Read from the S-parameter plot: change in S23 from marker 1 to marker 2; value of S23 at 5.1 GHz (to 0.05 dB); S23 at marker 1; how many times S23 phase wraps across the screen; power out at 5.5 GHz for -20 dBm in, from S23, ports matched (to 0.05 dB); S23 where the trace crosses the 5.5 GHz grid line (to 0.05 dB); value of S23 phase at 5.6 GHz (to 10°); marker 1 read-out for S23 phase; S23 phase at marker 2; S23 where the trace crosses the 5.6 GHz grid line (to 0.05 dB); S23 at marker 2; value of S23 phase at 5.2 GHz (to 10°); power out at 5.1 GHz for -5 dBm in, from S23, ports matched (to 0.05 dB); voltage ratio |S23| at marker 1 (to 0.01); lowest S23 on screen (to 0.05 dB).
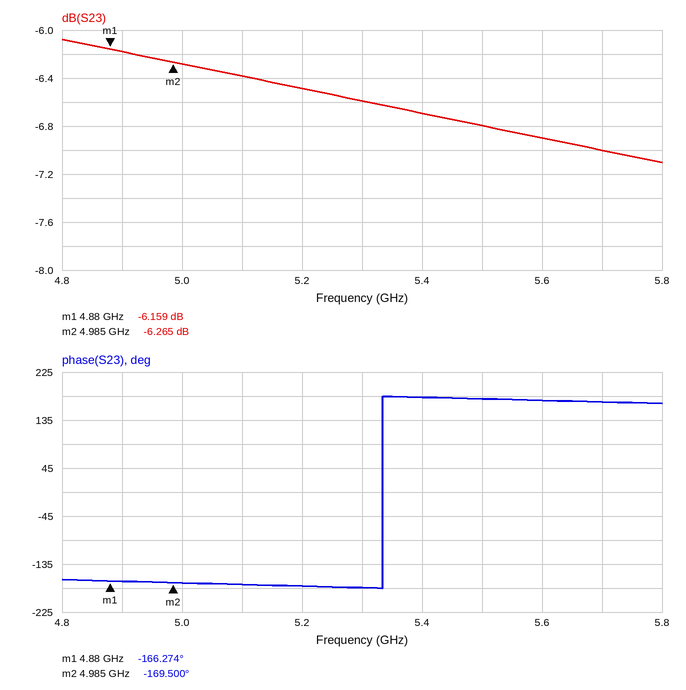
-0.106 dB
-6.40 dB
-6.159 dB
1
-26.80 dBm
-6.80 dB
170°
-166.274°
-169.500°
-6.90 dB
-6.265 dB
-180°
-11.40 dBm
0.49
-7.10 dB
